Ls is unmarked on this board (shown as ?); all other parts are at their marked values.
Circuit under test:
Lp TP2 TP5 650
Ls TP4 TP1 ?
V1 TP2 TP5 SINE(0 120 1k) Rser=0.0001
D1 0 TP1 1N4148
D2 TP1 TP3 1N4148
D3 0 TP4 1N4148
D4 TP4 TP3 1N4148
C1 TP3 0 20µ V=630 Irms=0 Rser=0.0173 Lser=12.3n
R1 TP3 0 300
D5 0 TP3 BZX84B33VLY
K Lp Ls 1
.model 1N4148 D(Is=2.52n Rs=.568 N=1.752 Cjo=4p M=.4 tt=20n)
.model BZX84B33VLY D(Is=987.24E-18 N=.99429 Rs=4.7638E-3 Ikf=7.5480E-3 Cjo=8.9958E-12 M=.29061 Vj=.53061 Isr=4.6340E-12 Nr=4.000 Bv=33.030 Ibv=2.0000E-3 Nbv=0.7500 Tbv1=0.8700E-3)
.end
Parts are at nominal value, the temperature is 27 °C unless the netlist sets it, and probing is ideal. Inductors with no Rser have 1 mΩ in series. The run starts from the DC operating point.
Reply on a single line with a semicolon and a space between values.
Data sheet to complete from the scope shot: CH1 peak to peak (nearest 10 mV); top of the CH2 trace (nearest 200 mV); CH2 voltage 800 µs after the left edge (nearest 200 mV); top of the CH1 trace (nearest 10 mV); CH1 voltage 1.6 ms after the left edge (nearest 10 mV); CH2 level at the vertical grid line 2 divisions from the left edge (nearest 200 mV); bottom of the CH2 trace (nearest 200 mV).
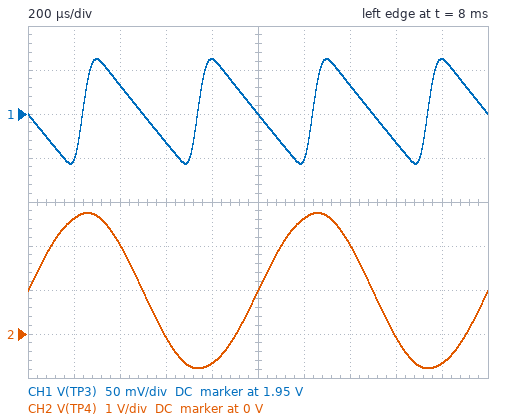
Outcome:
120 mV; 2.8 V; -600 mV; 2.01 V; 1.92 V; 2.0 V; -800 mV
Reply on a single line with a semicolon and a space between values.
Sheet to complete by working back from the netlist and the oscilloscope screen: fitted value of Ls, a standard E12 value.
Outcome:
560 mH
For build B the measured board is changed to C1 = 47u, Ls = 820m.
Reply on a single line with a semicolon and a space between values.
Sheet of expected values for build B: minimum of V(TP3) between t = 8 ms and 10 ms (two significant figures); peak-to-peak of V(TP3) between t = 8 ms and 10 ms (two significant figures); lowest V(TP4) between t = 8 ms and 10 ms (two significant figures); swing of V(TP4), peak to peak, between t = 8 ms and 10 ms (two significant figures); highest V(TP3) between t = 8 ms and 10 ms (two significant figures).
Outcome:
2.6 V; 70 mV; -810 mV; 4.3 V; 2.7 V
